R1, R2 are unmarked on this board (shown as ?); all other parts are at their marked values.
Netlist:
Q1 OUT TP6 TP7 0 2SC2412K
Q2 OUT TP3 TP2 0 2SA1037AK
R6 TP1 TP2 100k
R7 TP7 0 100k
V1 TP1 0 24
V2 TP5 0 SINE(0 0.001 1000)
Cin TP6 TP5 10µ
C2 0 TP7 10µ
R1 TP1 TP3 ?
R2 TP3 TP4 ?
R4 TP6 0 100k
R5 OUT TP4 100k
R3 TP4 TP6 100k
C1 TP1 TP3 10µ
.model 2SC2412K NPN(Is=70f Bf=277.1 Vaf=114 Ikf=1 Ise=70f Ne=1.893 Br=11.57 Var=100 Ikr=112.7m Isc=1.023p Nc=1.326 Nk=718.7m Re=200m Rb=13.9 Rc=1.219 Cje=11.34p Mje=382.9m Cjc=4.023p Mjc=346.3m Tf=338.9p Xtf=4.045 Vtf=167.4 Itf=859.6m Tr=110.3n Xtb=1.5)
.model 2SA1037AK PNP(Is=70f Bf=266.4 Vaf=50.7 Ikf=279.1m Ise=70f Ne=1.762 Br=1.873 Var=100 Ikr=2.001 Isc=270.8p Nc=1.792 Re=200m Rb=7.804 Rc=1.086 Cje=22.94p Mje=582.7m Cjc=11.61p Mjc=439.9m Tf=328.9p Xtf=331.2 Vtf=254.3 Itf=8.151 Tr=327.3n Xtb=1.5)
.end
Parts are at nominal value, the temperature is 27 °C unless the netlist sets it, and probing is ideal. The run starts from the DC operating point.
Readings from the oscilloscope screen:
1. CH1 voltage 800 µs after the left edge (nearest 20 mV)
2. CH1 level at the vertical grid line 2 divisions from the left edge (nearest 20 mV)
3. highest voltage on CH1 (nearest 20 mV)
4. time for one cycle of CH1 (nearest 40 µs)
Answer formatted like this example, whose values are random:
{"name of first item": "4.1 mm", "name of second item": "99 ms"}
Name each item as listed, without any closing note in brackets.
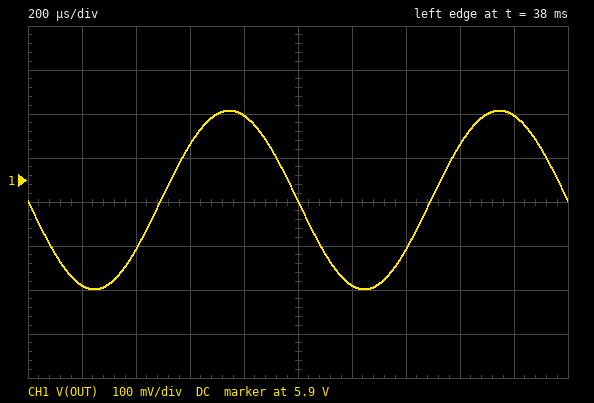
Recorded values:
{"CH1 voltage 800 µs after the left edge": "6.04 V", "CH1 level at the vertical grid line 2 divisions from the left edge": "5.74 V", "highest voltage on CH1": "6.06 V", "time for one cycle of CH1": "1.00 ms"}
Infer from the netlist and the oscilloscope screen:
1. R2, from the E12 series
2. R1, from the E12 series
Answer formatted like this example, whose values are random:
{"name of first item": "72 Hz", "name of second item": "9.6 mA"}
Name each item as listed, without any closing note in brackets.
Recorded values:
{"R2, from the E12 series": "270 kΩ", "R1, from the E12 series": "39 kΩ"}
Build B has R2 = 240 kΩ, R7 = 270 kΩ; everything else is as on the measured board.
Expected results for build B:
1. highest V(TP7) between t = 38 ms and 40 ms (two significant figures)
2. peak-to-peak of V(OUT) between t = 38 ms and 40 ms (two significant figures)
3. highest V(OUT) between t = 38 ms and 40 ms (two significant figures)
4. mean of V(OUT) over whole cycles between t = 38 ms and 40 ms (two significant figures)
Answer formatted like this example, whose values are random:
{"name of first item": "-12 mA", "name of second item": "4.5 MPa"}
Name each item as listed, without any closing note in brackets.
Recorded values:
{"highest V(TP7) between t = 38 ms and 40 ms": "4.4 V", "peak-to-peak of V(OUT) between t = 38 ms and 40 ms": "210 mV", "highest V(OUT) between t = 38 ms and 40 ms": "9.8 V", "mean of V(OUT) over whole cycles between t = 38 ms and 40 ms": "9.7 V"}
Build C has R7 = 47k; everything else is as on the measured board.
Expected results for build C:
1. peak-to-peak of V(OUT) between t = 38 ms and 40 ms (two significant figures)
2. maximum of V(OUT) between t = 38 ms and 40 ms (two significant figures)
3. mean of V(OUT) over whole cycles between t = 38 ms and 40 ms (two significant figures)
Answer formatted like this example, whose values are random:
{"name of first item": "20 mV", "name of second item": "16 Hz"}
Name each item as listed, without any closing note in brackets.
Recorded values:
{"peak-to-peak of V(OUT) between t = 38 ms and 40 ms": "470 mV", "maximum of V(OUT) between t = 38 ms and 40 ms": "2.9 V", "mean of V(OUT) over whole cycles between t = 38 ms and 40 ms": "2.6 V"}
